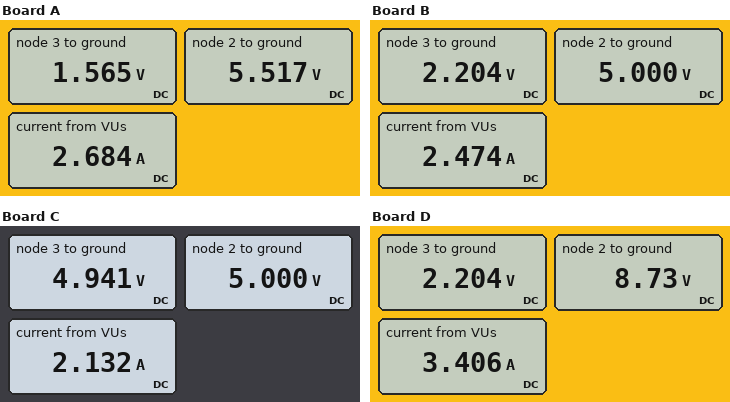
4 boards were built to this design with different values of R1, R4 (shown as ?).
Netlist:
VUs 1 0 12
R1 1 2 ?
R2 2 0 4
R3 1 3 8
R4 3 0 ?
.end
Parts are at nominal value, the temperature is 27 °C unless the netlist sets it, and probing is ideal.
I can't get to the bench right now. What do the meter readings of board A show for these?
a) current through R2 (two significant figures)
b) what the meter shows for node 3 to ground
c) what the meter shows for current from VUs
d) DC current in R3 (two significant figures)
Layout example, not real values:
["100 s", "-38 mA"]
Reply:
["1.4 A", "1.565 V", "2.684 A", "1.3 A"]
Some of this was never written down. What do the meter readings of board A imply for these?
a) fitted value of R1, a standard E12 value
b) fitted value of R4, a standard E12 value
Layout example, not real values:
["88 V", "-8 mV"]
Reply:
["4.7 Ω", "1.2 Ω"]
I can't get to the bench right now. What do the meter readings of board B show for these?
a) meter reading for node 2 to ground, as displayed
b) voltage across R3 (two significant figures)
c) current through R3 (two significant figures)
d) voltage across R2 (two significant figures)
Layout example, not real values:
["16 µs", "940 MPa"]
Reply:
["5.000 V", "9.8 V", "1.2 A", "5.0 V"]
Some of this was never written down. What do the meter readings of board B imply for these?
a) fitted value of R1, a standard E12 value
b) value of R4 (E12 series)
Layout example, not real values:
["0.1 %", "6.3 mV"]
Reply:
["5.6 Ω", "1.8 Ω"]
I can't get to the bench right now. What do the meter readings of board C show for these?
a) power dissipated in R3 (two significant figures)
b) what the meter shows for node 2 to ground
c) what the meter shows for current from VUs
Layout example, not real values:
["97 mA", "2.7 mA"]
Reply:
["6.2 W", "5.000 V", "2.132 A"]
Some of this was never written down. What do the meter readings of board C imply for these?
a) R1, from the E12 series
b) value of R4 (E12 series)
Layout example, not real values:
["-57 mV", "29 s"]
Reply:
["5.6 Ω", "5.6 Ω"]
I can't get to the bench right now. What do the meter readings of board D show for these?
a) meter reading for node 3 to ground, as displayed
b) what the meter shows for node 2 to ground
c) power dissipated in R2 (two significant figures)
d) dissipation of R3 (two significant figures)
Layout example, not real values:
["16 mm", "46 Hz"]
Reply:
["2.204 V", "8.73 V", "19 W", "12 W"]
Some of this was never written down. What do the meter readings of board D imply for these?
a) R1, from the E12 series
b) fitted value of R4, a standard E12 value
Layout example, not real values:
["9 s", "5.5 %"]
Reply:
["1.5 Ω", "1.8 Ω"]
